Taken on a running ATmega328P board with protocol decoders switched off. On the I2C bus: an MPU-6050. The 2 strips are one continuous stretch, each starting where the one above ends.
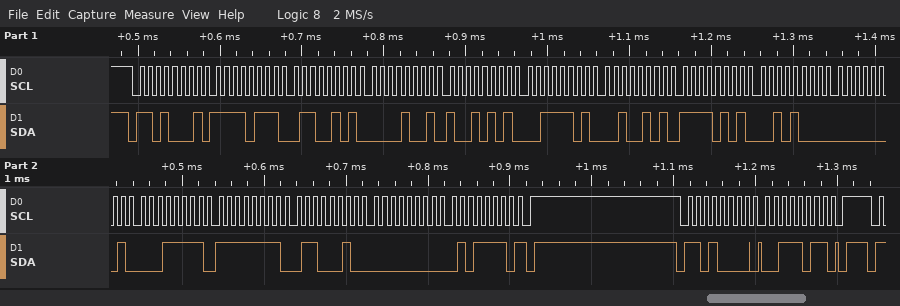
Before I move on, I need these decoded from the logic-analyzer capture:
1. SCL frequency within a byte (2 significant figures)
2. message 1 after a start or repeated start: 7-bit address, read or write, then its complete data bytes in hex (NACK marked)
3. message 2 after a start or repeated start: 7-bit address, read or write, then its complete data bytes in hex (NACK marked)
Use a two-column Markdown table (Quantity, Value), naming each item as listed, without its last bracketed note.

| Quantity | Value |
|---|---|
| SCL frequency within a byte | 100 kHz |
| message 1 after a start or repeated start: 7-bit address, read or write, then its complete data bytes in hex | 0x68 read: F7 65 09 95 3D 25 F5 28 01 1F FF 62 00 5E NACK |
| message 2 after a start or repeated start: 7-bit address, read or write, then its complete data bytes in hex | 0x68 write: 3B |
